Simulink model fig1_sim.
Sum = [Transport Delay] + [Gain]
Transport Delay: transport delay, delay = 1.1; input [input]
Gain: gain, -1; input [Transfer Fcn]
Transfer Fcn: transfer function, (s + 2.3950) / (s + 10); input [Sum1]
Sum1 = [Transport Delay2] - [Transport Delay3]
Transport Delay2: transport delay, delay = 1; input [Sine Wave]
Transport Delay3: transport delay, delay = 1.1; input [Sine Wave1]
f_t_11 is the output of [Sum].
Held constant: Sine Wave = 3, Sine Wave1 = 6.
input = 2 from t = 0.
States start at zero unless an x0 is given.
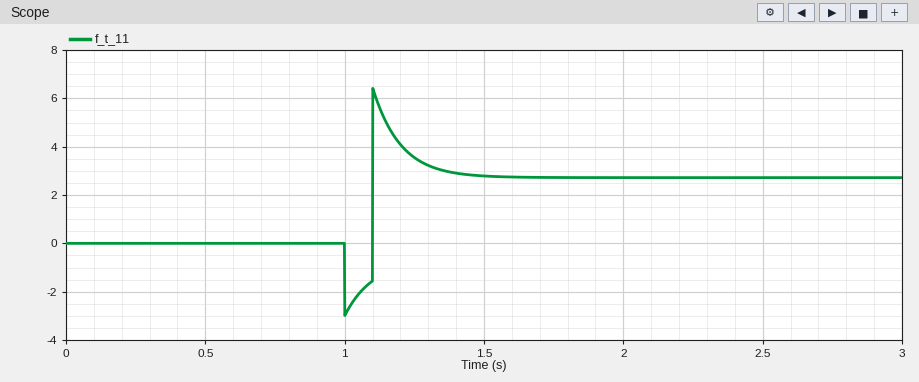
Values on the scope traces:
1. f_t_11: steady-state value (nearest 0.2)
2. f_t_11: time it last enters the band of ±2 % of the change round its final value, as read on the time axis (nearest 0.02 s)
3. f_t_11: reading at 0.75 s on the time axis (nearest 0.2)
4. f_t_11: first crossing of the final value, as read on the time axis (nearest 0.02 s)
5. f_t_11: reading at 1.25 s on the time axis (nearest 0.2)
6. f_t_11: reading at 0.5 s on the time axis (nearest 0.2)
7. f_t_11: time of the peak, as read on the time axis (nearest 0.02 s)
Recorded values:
2.8
1.52 s
0.0
1.10 s
3.6
0.0
1.10 s
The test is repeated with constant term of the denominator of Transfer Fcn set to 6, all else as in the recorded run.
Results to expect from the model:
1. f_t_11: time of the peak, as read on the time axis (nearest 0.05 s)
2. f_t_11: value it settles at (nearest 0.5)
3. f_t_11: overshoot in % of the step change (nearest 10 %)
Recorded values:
1.10 s
3.0
80 %
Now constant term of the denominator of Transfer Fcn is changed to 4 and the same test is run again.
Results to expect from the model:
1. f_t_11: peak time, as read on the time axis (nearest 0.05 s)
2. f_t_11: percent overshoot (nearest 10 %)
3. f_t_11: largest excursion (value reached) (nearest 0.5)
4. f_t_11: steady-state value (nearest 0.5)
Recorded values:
1.10 s
40 %
5.5
4.0
